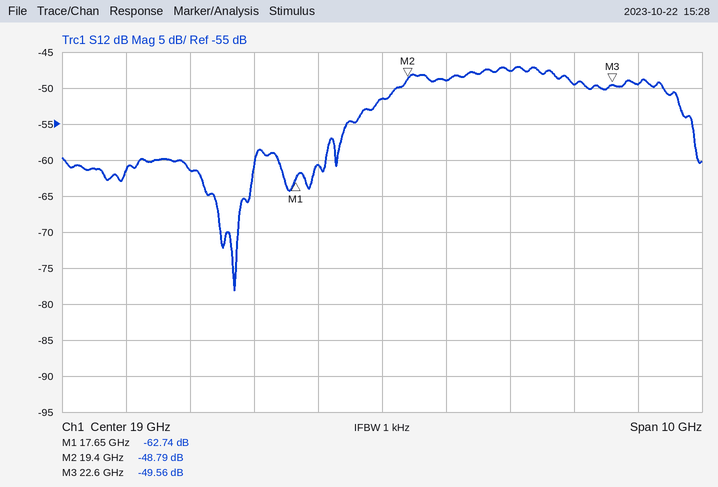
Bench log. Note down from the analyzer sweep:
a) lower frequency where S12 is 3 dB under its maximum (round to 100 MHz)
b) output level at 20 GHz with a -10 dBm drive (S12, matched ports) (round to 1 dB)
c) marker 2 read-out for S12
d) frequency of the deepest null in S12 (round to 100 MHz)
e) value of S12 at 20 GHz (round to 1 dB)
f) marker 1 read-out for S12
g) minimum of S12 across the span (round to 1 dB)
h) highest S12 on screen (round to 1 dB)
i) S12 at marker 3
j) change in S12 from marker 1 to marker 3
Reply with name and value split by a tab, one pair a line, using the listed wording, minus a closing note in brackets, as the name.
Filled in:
lower frequency where S12 is 3 dB under its maximum	19.2 GHz
output level at 20 GHz with a -10 dBm drive (S12, matched ports)	-59 dBm
marker 2 read-out for S12	-48.79 dB
frequency of the deepest null in S12	16.7 GHz
value of S12 at 20 GHz	-49 dB
marker 1 read-out for S12	-62.74 dB
minimum of S12 across the span	-78 dB
highest S12 on screen	-47 dB
S12 at marker 3	-49.56 dB
change in S12 from marker 1 to marker 3	13.18 dB
